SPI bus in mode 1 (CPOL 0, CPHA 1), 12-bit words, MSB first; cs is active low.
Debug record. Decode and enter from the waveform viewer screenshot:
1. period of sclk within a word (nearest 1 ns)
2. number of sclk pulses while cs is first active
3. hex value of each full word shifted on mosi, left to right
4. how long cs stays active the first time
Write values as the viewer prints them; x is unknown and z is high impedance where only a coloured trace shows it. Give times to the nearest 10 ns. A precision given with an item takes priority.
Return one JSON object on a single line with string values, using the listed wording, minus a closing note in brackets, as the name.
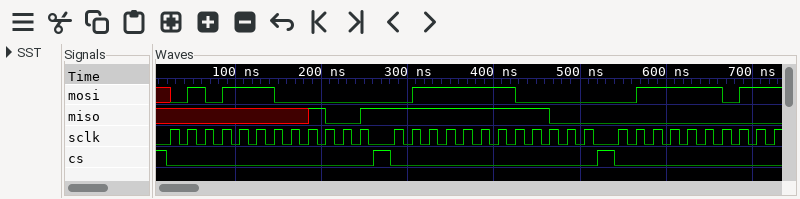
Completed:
{"period of sclk within a word": "20 ns", "number of sclk pulses while cs is first active": "12", "hex value of each full word shifted on mosi, left to right": "5C0, 7E0", "how long cs stays active the first time": "240 ns"}
